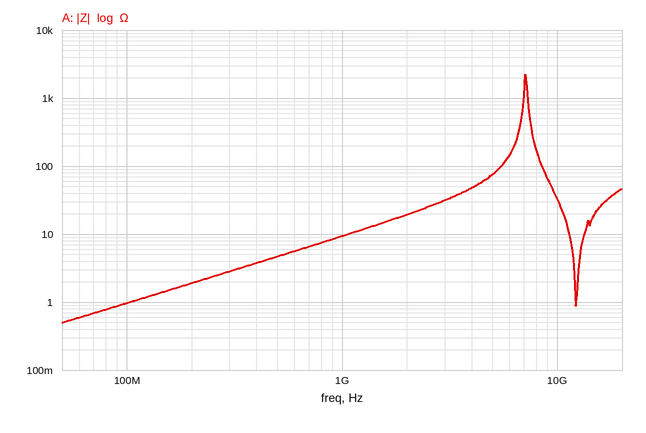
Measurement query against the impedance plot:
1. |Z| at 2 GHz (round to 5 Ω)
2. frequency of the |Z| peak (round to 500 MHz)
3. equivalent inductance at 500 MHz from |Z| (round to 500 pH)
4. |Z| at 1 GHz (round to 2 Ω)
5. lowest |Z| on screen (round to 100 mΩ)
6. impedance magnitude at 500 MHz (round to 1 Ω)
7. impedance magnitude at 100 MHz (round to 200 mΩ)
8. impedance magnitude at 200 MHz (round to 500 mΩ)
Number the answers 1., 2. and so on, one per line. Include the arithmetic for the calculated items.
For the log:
1. 20 Ω
2. 7.0 GHz
3. L = 5 Ω/(2π × 500 MHz) ≈ 1.59 nH, so 1.5 nH to the nearest 500 pH
4. 10 Ω
5. 500 mΩ
6. 5 Ω
7. 1.0 Ω
8. 2.0 Ω
